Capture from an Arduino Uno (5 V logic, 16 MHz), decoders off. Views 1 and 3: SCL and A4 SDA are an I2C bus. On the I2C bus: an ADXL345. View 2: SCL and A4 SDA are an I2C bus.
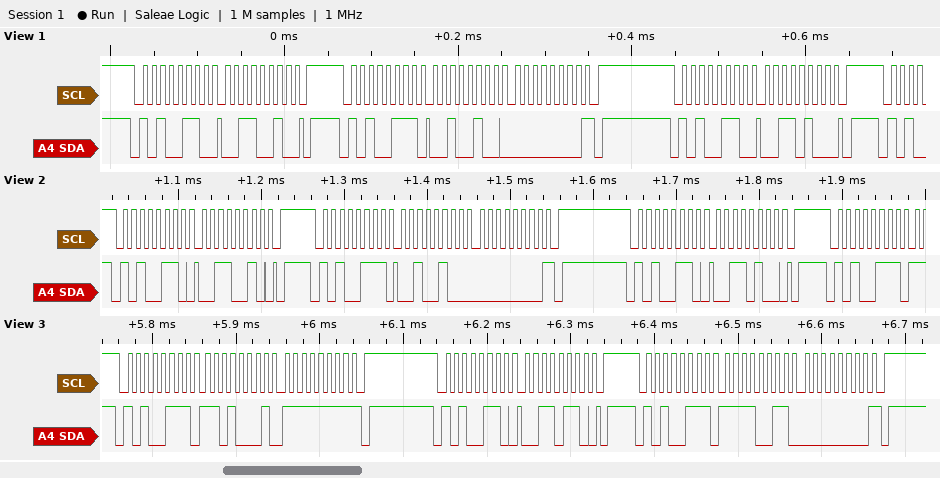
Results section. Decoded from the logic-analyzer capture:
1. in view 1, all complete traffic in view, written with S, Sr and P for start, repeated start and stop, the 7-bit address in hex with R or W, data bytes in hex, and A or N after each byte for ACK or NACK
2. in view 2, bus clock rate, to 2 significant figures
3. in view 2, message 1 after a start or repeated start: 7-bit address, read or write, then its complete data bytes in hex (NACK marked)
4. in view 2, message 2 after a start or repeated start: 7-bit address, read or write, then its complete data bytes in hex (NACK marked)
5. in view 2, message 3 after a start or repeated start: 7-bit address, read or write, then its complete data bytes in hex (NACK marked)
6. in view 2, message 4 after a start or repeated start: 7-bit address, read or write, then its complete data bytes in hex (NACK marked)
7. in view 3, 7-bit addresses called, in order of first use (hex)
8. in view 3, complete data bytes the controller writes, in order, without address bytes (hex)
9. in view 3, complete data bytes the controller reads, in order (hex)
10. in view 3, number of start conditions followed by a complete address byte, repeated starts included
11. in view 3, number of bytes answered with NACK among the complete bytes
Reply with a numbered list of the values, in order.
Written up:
1. S 53W A 32 A P S 53R A 24 A 00 N P S 53W A 34 A P
2. 100 kHz
3. 0x53 write: 32
4. 0x53 read: 24 00 NACK
5. 0x53 write: 34
6. 0x53 read
7. 0x53
8. 36
9. D1 FF F3 00
10. 3
11. 2
